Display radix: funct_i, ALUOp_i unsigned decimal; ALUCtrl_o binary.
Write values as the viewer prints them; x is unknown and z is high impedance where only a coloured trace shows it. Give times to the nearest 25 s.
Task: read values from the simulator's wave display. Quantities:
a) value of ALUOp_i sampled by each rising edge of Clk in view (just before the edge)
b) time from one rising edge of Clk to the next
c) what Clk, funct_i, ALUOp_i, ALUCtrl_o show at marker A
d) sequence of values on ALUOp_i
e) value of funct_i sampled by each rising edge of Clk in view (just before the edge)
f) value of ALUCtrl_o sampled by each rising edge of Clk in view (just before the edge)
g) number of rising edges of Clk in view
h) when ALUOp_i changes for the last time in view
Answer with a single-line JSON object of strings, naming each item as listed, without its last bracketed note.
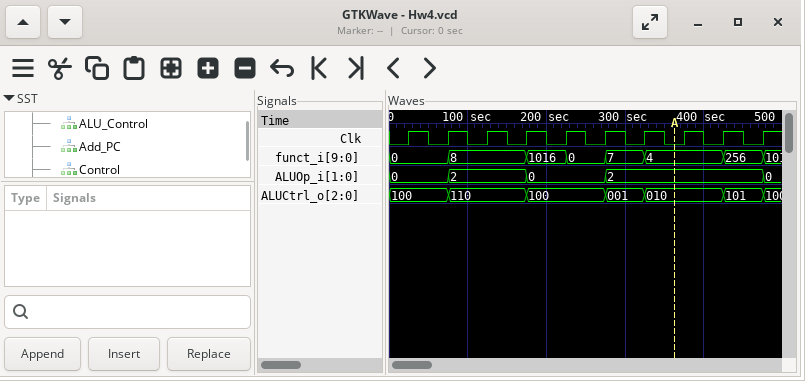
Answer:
{"value of ALUOp_i sampled by each rising edge of Clk in view": "0, 0, 2, 2, 0, 0, 2, 2, 2, 2", "time from one rising edge of Clk to the next": "50 s", "what Clk, funct_i, ALUOp_i, ALUCtrl_o show at marker A": "Clk=0, funct_i=4, ALUOp_i=2, ALUCtrl_o=010", "sequence of values on ALUOp_i": "0, 2, 0, 2, 0", "value of funct_i sampled by each rising edge of Clk in view": "0, 0, 8, 8, 1016, 0, 7, 4, 4, 256", "value of ALUCtrl_o sampled by each rising edge of Clk in view": "100, 100, 110, 110, 100, 100, 001, 010, 010, 101", "number of rising edges of Clk in view": "10", "when ALUOp_i changes for the last time in view": "475 s"}
